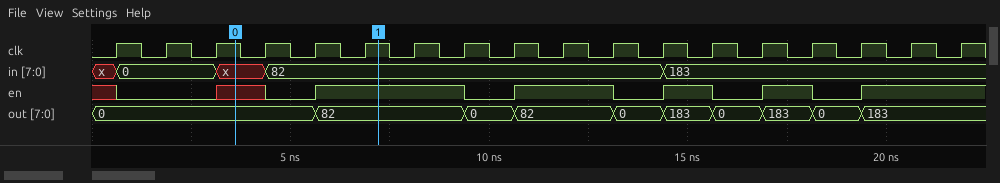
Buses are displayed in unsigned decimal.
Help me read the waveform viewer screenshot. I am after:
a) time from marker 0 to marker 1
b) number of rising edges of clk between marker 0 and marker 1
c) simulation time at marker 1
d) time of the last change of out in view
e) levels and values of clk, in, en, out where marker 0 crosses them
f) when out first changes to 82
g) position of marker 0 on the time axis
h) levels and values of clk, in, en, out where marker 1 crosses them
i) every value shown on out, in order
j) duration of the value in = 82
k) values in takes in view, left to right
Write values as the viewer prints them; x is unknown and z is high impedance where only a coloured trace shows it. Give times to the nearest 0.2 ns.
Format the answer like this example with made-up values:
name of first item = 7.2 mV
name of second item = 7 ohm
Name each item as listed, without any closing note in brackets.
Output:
time from marker 0 to marker 1 = 3.6 ns
number of rising edges of clk between marker 0 and marker 1 = 3
simulation time at marker 1 = 7.2 ns
time of the last change of out in view = 19.4 ns
levels and values of clk, in, en, out where marker 0 crosses them = clk=1, in=x, en=x, out=0
when out first changes to 82 = 5.6 ns
position of marker 0 on the time axis = 3.6 ns
levels and values of clk, in, en, out where marker 1 crosses them = clk=1, in=82, en=1, out=82
every value shown on out, in order = 0, 82, 0, 82, 0, 183, 0, 183, 0, 183
duration of the value in = 82 = 10 ns
values in takes in view, left to right = x, 0, x, 82, 183
